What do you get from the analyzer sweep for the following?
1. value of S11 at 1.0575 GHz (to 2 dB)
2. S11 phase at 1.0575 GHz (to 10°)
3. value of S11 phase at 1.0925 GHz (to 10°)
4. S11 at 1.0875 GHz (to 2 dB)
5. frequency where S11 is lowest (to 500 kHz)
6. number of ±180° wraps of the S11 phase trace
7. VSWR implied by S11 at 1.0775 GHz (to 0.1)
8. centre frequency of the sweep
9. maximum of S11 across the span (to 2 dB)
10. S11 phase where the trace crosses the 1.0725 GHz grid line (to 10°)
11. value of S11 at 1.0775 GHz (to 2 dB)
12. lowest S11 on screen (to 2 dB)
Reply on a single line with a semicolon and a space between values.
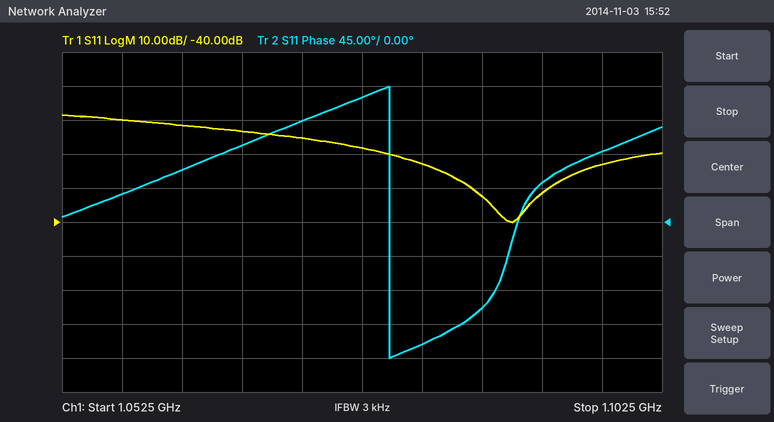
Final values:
-10 dB; 40°; 50°; -32 dB; 1.0900 GHz; 1; 1.3; 1.0775 GHz; -8 dB; 130°; -18 dB; -40 dB
